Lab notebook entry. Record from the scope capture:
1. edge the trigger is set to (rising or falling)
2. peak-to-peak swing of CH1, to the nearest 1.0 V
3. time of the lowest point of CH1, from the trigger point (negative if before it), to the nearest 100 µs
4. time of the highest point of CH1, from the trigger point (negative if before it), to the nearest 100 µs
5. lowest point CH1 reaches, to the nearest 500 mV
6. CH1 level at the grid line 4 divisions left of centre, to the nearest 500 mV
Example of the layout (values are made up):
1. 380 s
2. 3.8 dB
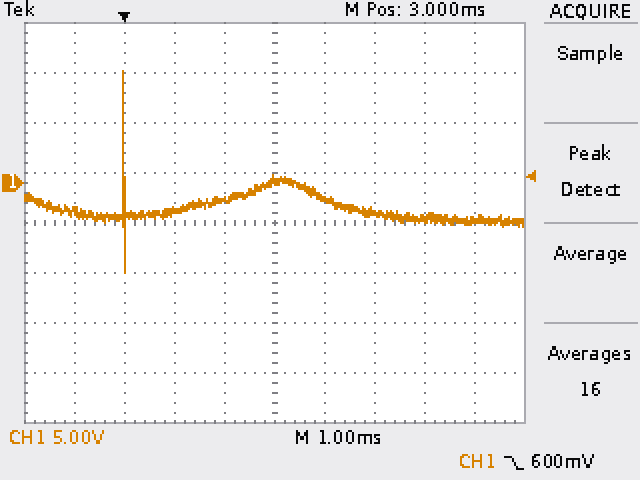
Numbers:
1. falling
2. 20.0 V
3. 0.0 ms
4. 0.0 ms
5. -9.0 V
6. -3.0 V
